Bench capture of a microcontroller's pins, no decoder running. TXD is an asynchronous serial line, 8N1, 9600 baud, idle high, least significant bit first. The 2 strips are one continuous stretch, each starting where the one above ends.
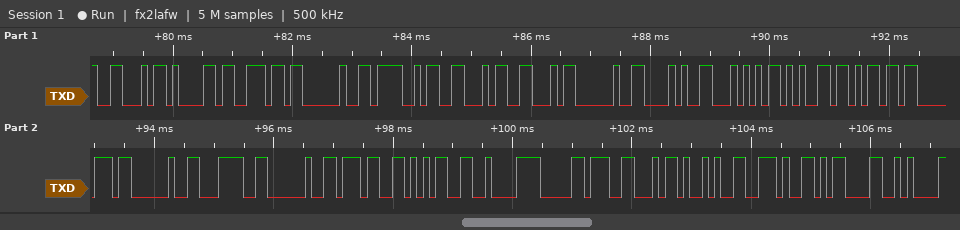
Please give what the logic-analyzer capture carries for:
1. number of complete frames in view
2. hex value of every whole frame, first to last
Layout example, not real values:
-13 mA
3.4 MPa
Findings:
25
46 61 6E 20 4F 46 46 20 28 54 65 6D 70 20 3C 20 37 35 C2 B0 46 29 2E 0D 0A
